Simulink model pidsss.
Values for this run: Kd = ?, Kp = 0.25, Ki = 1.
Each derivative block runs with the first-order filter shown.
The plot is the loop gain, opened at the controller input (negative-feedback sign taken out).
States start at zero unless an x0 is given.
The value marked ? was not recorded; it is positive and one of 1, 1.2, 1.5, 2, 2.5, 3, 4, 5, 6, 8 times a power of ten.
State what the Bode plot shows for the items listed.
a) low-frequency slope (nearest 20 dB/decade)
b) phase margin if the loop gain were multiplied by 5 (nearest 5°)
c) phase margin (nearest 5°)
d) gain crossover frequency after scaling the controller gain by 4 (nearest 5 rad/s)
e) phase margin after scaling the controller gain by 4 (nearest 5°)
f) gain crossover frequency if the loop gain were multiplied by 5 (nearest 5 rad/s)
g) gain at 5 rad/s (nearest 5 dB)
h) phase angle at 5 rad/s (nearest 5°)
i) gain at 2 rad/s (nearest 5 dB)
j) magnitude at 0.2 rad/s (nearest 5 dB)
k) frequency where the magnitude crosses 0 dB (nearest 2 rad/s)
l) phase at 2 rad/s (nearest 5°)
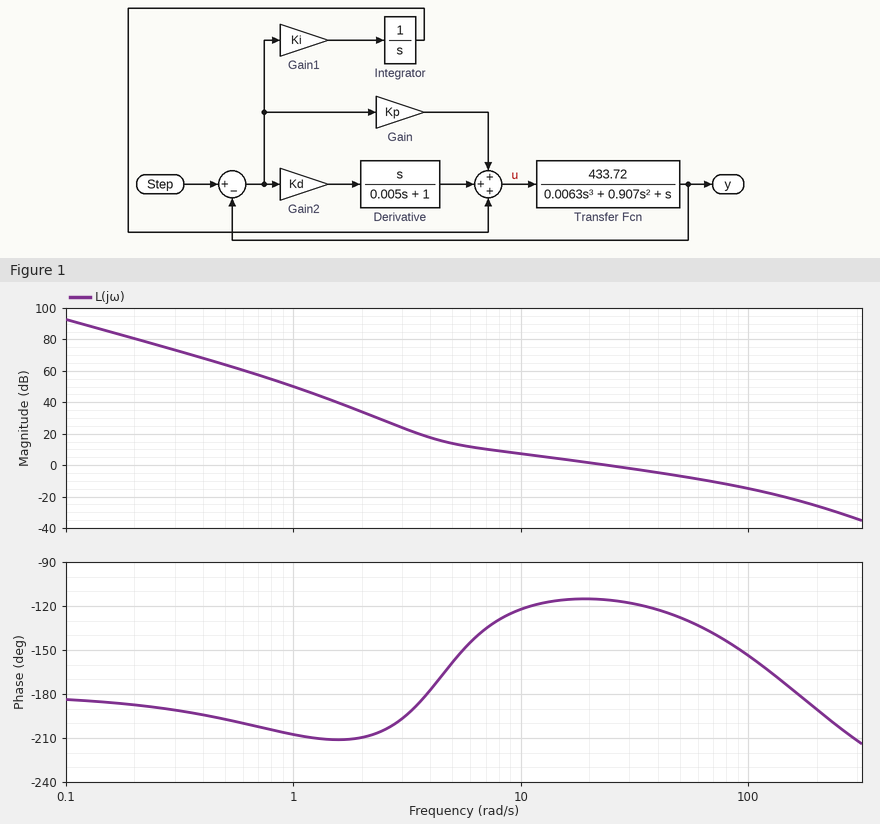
-40 dB/decade
30°
65°
80 rad/s
35°
95 rad/s
15 dB
-160°
35 dB
80 dB
24 rad/s
-210°
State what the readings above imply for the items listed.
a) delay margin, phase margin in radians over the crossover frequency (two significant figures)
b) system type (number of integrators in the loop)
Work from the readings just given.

0.047 s
2
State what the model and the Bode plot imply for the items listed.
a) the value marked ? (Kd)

0.05
